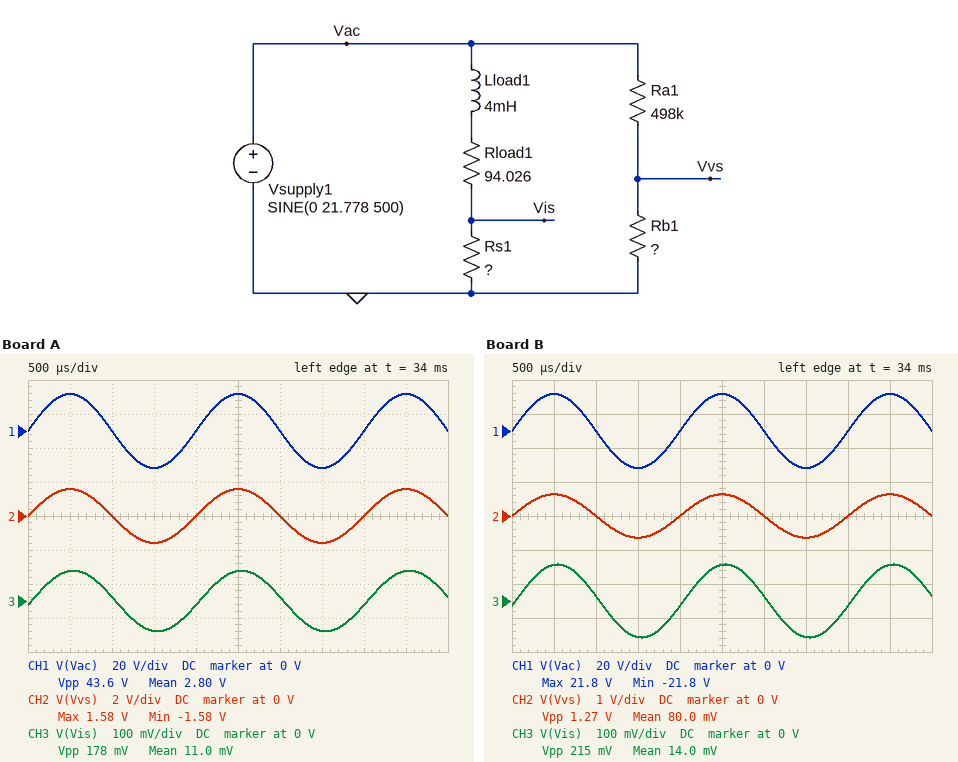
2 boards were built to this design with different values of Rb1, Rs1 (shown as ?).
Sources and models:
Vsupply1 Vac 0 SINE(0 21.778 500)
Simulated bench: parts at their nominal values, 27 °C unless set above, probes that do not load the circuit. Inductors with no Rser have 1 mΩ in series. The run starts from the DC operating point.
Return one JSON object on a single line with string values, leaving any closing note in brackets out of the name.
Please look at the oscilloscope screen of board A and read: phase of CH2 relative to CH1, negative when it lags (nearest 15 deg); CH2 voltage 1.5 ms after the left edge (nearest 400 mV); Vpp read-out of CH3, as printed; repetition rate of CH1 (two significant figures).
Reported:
{"phase of CH2 relative to CH1, negative when it lags": "0 deg", "CH2 voltage 1.5 ms after the left edge": "-1.6 V", "Vpp read-out of CH3, as printed": "178 mV", "repetition rate of CH1": "500 Hz"}
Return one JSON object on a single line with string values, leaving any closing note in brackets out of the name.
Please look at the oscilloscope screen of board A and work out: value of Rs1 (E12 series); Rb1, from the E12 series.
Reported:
{"value of Rs1": "0.39 Ω", "Rb1, from the E12 series": "39 kΩ"}
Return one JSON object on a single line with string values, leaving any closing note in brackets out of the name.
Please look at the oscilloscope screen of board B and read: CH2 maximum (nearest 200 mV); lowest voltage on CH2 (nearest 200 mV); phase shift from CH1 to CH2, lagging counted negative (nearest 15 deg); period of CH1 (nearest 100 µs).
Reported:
{"CH2 maximum": "600 mV", "lowest voltage on CH2": "-600 mV", "phase shift from CH1 to CH2, lagging counted negative": "0 deg", "period of CH1": "2.0 ms"}
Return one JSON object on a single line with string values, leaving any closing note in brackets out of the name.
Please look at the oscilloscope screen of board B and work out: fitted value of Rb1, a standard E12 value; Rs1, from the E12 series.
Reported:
{"fitted value of Rb1, a standard E12 value": "15 kΩ", "Rs1, from the E12 series": "0.47 Ω"}
